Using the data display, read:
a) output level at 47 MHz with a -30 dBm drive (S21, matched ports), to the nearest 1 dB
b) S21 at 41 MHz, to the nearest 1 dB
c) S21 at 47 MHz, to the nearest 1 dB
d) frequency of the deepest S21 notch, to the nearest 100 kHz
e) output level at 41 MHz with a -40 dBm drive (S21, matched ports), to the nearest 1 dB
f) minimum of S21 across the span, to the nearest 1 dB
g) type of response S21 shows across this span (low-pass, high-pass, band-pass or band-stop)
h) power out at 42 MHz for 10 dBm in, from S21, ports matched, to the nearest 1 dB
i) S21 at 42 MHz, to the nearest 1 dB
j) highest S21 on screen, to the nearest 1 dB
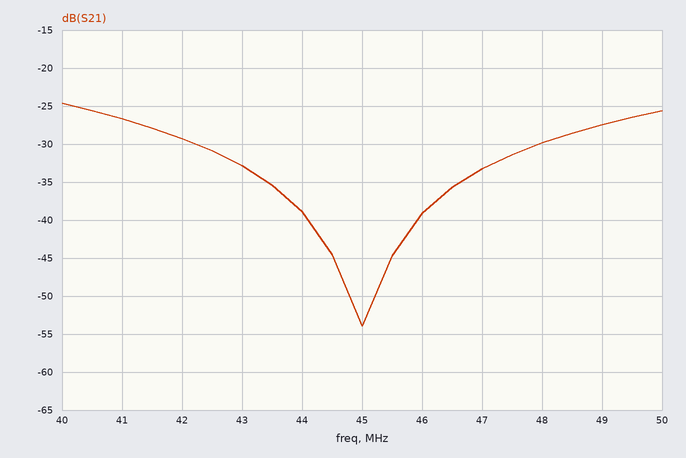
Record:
-63 dBm
-27 dB
-33 dB
45.0 MHz
-67 dBm
-54 dB
band-stop
-19 dBm
-29 dB
-25 dB
